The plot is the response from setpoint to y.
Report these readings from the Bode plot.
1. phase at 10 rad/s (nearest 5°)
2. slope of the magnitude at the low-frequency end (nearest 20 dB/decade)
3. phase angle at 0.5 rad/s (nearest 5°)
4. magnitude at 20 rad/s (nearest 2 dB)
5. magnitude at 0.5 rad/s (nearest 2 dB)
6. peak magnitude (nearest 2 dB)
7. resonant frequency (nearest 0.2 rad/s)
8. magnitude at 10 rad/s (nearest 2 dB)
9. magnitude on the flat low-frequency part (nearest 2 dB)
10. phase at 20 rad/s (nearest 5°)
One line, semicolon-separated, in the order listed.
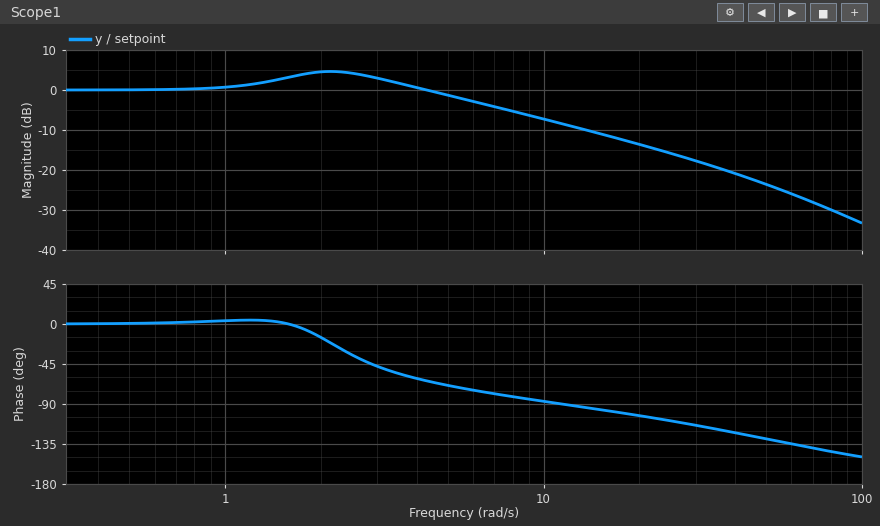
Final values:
-85°; 0 dB/decade; 0°; -14 dB; 0 dB; 4 dB; 2.2 rad/s; -8 dB; 0 dB; -105°
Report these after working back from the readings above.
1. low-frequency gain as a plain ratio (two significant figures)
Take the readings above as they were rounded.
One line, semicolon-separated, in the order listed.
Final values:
1.0
